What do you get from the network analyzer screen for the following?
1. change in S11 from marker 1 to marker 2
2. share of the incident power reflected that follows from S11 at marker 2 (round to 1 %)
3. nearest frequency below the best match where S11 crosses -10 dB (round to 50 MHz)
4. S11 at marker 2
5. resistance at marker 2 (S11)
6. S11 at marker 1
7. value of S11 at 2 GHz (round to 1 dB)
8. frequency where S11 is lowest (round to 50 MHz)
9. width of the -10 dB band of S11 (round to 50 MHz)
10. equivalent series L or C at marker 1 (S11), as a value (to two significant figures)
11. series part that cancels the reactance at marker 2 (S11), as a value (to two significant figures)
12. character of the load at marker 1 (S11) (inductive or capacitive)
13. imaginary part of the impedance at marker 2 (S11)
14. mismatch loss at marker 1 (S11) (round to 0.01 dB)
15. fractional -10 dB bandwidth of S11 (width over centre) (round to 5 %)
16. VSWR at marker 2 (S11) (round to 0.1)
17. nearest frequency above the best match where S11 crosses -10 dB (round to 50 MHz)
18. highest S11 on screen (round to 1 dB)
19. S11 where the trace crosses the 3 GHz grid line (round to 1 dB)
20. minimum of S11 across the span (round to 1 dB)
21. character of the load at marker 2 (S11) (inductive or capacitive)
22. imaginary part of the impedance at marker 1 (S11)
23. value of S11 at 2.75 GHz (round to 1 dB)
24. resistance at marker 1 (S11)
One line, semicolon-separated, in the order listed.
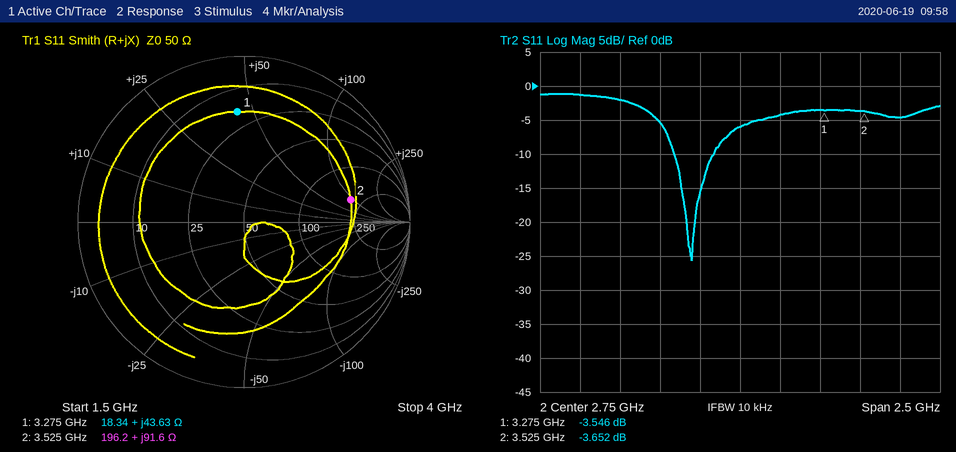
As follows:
-0.106 dB; 43 %; 2.35 GHz; -3.652 dB; 196.2 Ω; -3.546 dB; -2 dB; 2.45 GHz; 250 MHz; 2.1 nH; 490 fF; inductive; +91.6 Ω; 2.53 dB; 10 %; 4.8; 2.60 GHz; -1 dB; -4 dB; -26 dB; inductive; +43.63 Ω; -6 dB; 18.34 Ω
